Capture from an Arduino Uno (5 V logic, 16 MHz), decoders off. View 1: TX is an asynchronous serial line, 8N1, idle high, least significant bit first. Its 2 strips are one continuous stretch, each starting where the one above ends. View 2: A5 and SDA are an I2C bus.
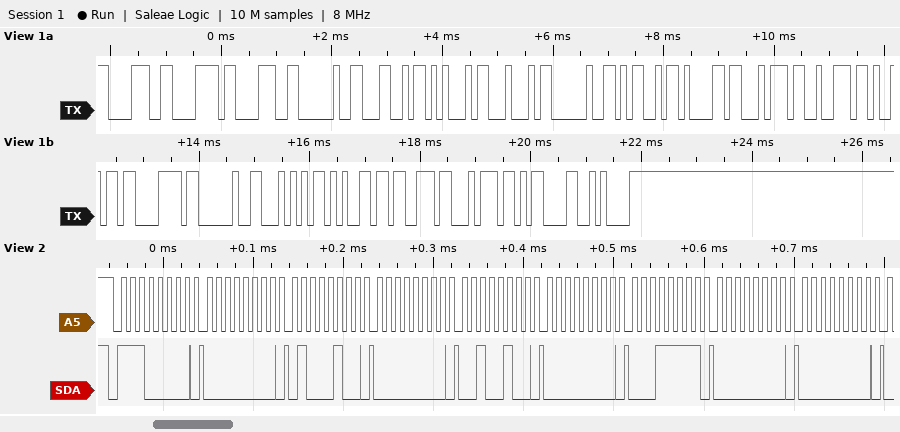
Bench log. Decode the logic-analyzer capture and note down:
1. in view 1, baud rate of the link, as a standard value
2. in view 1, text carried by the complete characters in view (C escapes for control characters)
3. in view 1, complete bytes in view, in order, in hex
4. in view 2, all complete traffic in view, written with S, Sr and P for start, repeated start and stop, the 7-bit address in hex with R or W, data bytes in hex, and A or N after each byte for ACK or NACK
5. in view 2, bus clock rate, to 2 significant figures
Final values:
9600 baud
"8x8 LED Matrix Test\r\n"
38 78 38 20 4C 45 44 20 4D 61 74 72 69 78 20 54 65 73 74 0D 0A
S 70W A 00 A 44 A 00 A 24 A 00 A 1F A 00 A 00 A
100 kHz
